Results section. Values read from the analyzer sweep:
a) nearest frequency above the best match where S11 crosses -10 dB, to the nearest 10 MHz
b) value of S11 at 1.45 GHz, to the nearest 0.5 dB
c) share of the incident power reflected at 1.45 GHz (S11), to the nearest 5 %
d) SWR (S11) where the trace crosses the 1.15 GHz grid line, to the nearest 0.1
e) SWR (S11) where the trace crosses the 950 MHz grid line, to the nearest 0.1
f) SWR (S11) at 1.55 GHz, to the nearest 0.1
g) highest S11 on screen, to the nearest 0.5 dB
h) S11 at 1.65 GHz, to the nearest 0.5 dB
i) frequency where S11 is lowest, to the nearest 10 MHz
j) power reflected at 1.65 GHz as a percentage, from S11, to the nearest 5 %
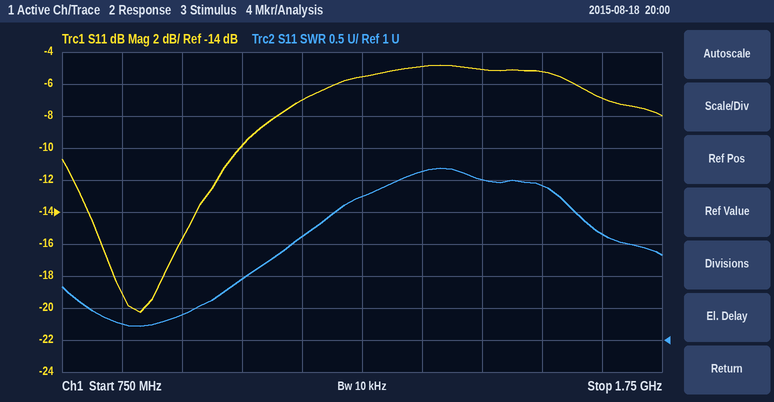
1.05 GHz
-5.0 dB
30 %
2.6
1.4
3.4
-5.0 dB
-7.0 dB
880 MHz
20 %
